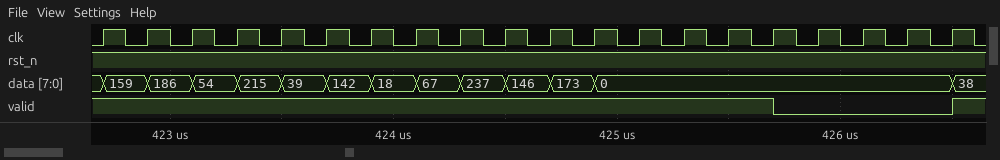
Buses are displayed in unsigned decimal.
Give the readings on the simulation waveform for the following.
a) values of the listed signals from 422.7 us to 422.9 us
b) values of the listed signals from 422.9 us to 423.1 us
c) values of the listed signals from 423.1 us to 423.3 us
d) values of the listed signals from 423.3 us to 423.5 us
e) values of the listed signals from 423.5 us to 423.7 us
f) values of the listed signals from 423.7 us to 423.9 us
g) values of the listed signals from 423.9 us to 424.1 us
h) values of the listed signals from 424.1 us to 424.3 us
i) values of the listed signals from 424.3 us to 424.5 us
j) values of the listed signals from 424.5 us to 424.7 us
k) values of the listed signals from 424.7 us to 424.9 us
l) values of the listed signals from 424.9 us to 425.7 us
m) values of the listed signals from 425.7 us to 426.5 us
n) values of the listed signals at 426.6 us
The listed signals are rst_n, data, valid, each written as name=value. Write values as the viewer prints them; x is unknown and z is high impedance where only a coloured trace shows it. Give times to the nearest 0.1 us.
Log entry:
rst_n=1, data=159, valid=1
rst_n=1, data=186, valid=1
rst_n=1, data=54, valid=1
rst_n=1, data=215, valid=1
rst_n=1, data=39, valid=1
rst_n=1, data=142, valid=1
rst_n=1, data=18, valid=1
rst_n=1, data=67, valid=1
rst_n=1, data=237, valid=1
rst_n=1, data=146, valid=1
rst_n=1, data=173, valid=1
rst_n=1, data=0, valid=1
rst_n=1, data=0, valid=0
rst_n=1, data=38, valid=1
